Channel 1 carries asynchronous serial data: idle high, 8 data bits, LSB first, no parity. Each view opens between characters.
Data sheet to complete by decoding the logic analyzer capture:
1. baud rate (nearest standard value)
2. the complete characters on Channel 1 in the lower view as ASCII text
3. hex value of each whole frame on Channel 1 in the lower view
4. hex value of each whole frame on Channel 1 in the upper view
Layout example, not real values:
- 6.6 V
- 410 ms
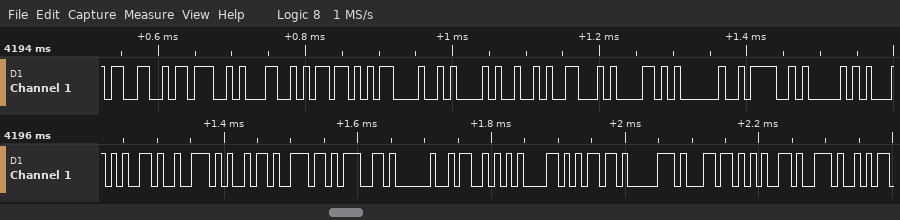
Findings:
- 115200 baud
- "ering Sample."
- 65, 72, 69, 6E, 67, 20, 53, 61, 6D, 70, 6C, 65, 2E
- 33, 3B, 31, 6D, 0D, 0A, 49, 46, 58, 20, 4F, 50
